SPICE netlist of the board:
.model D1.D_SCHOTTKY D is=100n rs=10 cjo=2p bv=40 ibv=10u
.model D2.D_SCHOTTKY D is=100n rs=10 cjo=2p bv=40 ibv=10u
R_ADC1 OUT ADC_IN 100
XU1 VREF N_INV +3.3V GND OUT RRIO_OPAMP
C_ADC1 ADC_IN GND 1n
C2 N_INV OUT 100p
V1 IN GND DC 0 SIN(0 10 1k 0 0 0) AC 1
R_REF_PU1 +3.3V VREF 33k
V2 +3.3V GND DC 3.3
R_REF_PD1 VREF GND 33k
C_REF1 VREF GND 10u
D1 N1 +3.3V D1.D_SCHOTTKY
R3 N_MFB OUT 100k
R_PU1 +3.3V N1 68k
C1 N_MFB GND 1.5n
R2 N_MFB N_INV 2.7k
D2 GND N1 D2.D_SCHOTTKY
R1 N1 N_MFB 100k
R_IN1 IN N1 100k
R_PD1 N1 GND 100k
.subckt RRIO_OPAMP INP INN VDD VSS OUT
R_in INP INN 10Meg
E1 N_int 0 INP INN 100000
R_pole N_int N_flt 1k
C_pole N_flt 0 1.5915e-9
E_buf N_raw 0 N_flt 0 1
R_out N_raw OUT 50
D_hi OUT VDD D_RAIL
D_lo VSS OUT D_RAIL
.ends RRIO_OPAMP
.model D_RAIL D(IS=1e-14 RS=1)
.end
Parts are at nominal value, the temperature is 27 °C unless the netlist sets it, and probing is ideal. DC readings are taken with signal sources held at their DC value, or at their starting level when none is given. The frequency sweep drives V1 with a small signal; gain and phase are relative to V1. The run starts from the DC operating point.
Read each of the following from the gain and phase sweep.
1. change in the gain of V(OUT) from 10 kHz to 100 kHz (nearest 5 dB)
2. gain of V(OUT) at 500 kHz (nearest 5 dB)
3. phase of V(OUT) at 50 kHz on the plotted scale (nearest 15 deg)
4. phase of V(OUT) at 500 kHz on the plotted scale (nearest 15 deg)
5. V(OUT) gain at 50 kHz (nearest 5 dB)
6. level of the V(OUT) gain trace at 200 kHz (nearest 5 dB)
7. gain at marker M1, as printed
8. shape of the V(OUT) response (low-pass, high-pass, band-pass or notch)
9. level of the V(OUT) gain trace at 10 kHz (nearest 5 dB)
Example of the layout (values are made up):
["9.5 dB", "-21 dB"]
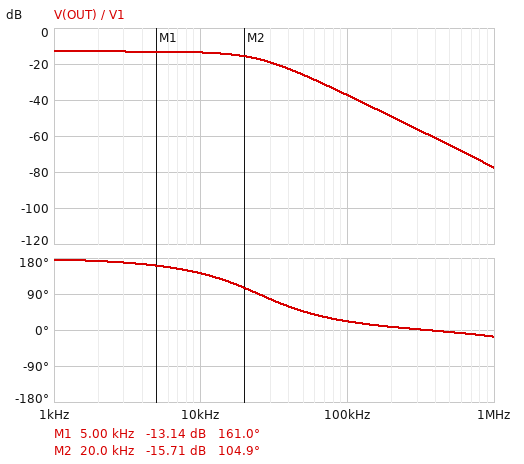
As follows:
["-25 dB", "-65 dB", "45 deg", "0 deg", "-25 dB", "-50 dB", "-13.14 dB", "low-pass", "-15 dB"]
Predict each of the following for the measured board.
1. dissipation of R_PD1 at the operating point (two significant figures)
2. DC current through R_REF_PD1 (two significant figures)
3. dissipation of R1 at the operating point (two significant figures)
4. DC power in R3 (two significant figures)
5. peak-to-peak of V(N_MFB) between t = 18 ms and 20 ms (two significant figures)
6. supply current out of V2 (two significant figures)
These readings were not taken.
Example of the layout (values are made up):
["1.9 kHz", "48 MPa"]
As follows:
["21 µW", "50 µA", "380 nW", "380 nW", "7.6 mV", "77 µA"]
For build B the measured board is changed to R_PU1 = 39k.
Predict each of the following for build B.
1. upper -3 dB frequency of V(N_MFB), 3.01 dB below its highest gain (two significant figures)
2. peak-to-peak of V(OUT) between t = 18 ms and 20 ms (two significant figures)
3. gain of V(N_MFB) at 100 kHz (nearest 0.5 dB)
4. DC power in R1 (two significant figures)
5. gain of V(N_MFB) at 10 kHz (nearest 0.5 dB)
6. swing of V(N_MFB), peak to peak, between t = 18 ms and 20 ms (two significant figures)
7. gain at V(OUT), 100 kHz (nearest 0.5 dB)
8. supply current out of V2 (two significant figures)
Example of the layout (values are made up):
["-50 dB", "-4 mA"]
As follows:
["53 kHz", "3.4 V", "-54.5 dB", "280 nW", "-51.0 dB", "6.1 mV", "-39.0 dB", "88 µA"]
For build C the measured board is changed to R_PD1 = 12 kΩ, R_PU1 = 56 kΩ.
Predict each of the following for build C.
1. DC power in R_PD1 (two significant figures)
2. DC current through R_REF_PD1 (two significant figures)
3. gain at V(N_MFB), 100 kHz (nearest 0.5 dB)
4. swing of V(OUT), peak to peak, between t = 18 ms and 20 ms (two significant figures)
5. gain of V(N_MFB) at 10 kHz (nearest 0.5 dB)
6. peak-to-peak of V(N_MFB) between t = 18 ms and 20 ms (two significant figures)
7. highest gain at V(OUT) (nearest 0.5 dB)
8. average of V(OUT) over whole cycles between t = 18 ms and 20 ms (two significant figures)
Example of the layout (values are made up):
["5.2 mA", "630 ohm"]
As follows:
["32 µW", "50 µA", "-61.5 dB", "1.6 V", "-57.5 dB", "2.8 mV", "-21.5 dB", "2.7 V"]
